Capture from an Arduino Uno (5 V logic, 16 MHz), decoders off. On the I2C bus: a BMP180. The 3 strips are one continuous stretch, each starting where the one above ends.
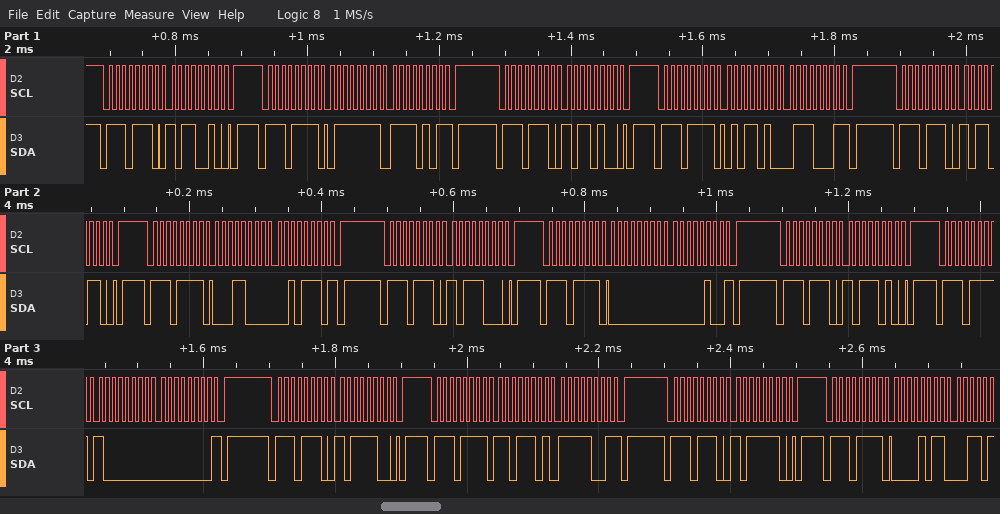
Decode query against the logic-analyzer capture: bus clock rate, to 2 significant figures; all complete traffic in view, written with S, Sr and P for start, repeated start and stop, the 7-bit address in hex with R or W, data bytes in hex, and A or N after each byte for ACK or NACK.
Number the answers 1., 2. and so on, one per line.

1. 100 kHz
2. S 77W A B2 A P S 77R A 7F A F5 N P S 77W A B4 A P S 77R A 5A A 71 N P S 77W A B6 A P S 77R A 18 A 2E N P S 77W A B8 A P S 77R A 00 A 04 N P S 77W A BA A P S 77R A 80 A 00 N P S 77W A BC A P S 77R A DD A F9 N P S 77W A BE A P S 77R A 0B A
